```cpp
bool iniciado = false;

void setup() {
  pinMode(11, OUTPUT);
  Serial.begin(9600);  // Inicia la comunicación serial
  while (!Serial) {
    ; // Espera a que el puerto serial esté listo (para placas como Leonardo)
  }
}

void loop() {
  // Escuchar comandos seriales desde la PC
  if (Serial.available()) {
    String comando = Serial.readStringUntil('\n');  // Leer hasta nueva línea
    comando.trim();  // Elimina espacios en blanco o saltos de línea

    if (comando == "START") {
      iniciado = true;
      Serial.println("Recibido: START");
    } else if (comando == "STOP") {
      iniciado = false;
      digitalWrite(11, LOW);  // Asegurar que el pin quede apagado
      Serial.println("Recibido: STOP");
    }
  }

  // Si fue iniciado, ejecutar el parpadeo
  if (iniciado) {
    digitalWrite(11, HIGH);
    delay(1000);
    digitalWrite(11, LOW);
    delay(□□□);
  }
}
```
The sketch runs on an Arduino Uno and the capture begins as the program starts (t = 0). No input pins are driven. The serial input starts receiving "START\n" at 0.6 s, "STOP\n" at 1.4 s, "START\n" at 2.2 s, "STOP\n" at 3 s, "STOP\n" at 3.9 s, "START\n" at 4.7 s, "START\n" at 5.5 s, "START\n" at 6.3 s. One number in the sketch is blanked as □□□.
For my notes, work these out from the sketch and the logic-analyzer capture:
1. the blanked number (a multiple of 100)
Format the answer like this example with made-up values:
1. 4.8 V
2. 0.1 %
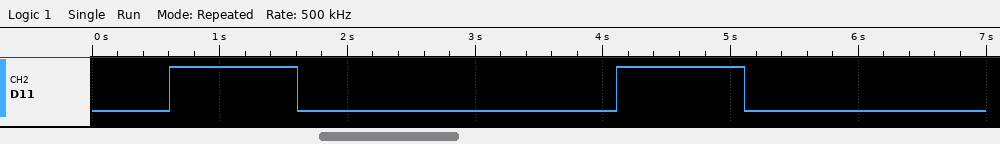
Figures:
1. 2500
